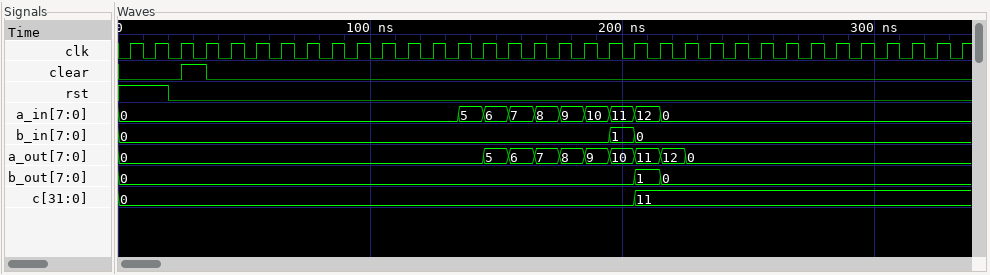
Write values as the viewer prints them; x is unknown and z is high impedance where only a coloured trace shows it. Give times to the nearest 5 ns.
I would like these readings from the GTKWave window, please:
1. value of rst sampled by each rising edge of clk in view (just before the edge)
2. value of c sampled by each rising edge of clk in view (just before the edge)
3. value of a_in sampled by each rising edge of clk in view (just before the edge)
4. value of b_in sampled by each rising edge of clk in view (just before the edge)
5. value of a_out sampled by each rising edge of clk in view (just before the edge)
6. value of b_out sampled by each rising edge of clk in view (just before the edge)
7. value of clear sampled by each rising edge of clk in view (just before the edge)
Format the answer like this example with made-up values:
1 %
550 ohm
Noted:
1 1 0 0 0 0 0 0 0 0 0 0 0 0 0 0 0 0 0 0 0 0 0 0 0 0 0 0 0 0 0 0 0 0
0, 0, 0, 0, 0, 0, 0, 0, 0, 0, 0, 0, 0, 0, 0, 0, 0, 0, 0, 0, 0, 11, 11, 11, 11, 11, 11, 11, 11, 11, 11, 11, 11, 11
0, 0, 0, 0, 0, 0, 0, 0, 0, 0, 0, 0, 0, 0, 5, 6, 7, 8, 9, 10, 11, 12, 0, 0, 0, 0, 0, 0, 0, 0, 0, 0, 0, 0
0, 0, 0, 0, 0, 0, 0, 0, 0, 0, 0, 0, 0, 0, 0, 0, 0, 0, 0, 0, 1, 0, 0, 0, 0, 0, 0, 0, 0, 0, 0, 0, 0, 0
0, 0, 0, 0, 0, 0, 0, 0, 0, 0, 0, 0, 0, 0, 0, 5, 6, 7, 8, 9, 10, 11, 12, 0, 0, 0, 0, 0, 0, 0, 0, 0, 0, 0
0, 0, 0, 0, 0, 0, 0, 0, 0, 0, 0, 0, 0, 0, 0, 0, 0, 0, 0, 0, 0, 1, 0, 0, 0, 0, 0, 0, 0, 0, 0, 0, 0, 0
0 0 0 1 0 0 0 0 0 0 0 0 0 0 0 0 0 0 0 0 0 0 0 0 0 0 0 0 0 0 0 0 0 0
